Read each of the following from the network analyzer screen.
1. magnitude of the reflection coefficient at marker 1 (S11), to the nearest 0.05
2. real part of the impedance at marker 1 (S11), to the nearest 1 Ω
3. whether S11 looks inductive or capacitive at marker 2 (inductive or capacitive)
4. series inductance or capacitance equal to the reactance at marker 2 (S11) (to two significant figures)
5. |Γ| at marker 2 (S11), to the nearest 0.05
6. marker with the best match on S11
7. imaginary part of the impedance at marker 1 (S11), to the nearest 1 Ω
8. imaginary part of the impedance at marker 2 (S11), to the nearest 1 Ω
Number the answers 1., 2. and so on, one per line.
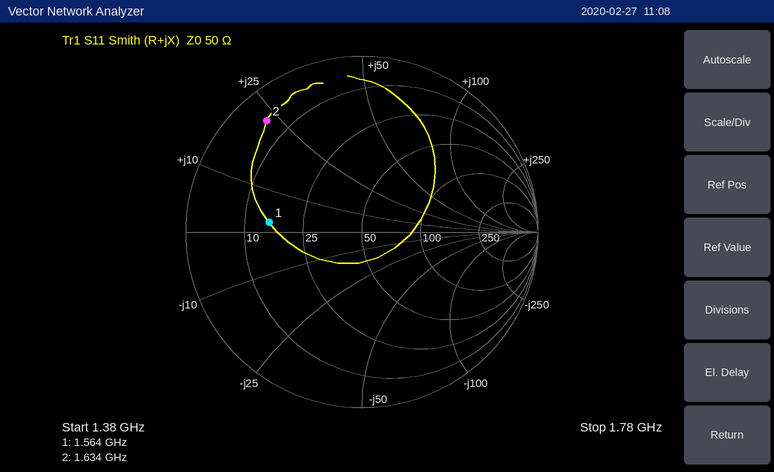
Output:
1. 0.55
2. 15 Ω
3. inductive
4. 2.2 nH
5. 0.85
6. marker 1
7. +2 Ω
8. +23 Ω
